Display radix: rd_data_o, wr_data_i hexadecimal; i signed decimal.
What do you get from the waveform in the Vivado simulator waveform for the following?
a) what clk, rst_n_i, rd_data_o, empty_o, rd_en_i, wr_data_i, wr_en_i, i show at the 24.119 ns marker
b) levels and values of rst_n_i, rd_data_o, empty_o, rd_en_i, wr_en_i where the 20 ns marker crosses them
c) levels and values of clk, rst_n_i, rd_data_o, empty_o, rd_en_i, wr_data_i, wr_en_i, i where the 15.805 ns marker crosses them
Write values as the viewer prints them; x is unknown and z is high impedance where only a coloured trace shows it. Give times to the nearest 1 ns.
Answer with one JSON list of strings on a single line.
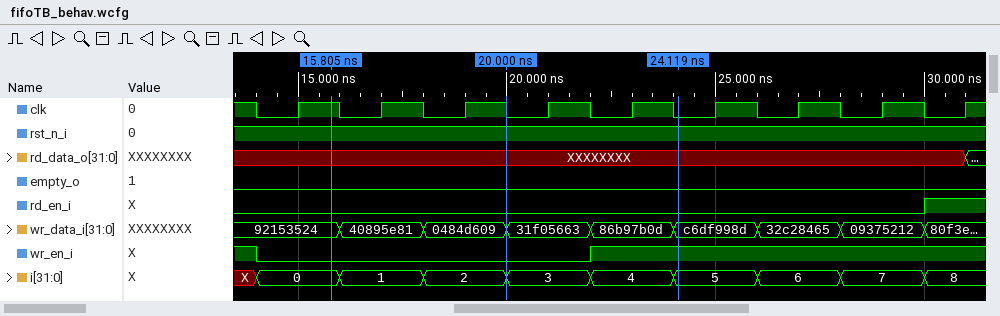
["clk=0, rst_n_i=1, rd_data_o=XXXXXXXX, empty_o=0, rd_en_i=0, wr_data_i=c6df998d, wr_en_i=1, i=5", "rst_n_i=1, rd_data_o=XXXXXXXX, empty_o=0, rd_en_i=0, wr_en_i=0", "clk=1, rst_n_i=1, rd_data_o=XXXXXXXX, empty_o=0, rd_en_i=0, wr_data_i=92153524, wr_en_i=0, i=0"]
